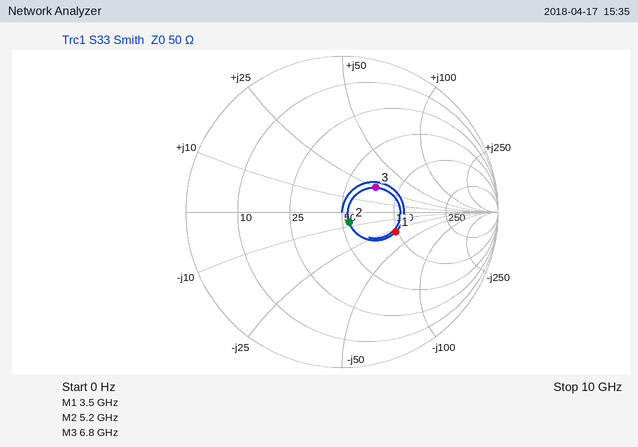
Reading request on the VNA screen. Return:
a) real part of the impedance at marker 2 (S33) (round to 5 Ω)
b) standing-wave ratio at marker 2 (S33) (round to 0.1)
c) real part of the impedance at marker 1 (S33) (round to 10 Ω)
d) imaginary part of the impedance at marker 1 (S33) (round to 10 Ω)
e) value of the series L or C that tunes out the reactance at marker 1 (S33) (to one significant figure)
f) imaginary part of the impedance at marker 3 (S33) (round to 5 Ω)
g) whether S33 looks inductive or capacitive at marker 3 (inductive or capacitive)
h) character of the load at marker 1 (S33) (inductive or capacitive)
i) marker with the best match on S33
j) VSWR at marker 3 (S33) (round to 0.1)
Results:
55 Ω
1.2
100 Ω
-30 Ω
1 nH
+25 Ω
inductive
capacitive
marker 2
1.7
